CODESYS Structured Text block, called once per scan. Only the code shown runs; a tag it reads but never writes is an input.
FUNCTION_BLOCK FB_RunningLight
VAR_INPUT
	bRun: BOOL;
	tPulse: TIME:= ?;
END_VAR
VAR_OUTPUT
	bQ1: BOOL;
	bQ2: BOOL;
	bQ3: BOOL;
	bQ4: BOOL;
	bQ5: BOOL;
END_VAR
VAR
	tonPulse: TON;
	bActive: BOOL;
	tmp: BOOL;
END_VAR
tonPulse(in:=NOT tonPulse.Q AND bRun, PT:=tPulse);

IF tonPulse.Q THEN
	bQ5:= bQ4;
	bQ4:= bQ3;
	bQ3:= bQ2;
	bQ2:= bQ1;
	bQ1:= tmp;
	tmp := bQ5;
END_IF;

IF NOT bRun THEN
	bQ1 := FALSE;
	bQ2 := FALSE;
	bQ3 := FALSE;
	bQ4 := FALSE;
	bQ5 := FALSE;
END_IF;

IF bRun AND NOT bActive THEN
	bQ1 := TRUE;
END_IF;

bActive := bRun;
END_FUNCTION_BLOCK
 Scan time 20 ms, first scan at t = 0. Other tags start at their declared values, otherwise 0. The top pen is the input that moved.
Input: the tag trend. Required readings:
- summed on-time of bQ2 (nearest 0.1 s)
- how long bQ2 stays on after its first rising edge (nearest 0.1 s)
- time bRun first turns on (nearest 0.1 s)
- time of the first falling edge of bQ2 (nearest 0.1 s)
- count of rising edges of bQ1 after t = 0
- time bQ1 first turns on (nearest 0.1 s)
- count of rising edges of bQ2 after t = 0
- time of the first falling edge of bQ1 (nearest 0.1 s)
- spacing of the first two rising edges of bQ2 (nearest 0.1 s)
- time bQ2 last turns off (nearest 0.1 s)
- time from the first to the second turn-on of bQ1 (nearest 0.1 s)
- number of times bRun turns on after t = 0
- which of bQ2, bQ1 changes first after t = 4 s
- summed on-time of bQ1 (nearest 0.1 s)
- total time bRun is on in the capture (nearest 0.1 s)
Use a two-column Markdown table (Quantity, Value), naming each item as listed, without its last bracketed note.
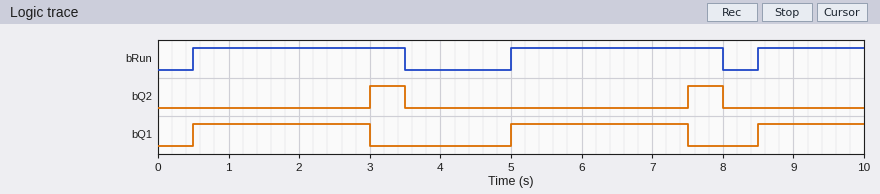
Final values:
| Quantity | Value |
|---|---|
| summed on-time of bQ2 | 1.0 s |
| how long bQ2 stays on after its first rising edge | 0.5 s |
| time bRun first turns on | 0.5 s |
| time of the first falling edge of bQ2 | 3.5 s |
| count of rising edges of bQ1 after t = 0 | 3 |
| time bQ1 first turns on | 0.5 s |
| count of rising edges of bQ2 after t = 0 | 2 |
| time of the first falling edge of bQ1 | 3.0 s |
| spacing of the first two rising edges of bQ2 | 4.5 s |
| time bQ2 last turns off | 8.0 s |
| time from the first to the second turn-on of bQ1 | 4.5 s |
| number of times bRun turns on after t = 0 | 3 |
| which of bQ2, bQ1 changes first after t = 4 s | bQ1 |
| summed on-time of bQ1 | 6.5 s |
| total time bRun is on in the capture | 7.5 s |
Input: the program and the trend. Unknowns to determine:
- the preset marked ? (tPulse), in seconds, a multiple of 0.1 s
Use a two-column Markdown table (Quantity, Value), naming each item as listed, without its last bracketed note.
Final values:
| Quantity | Value |
|---|---|
| the preset marked ? (tPulse), in seconds, a multiple of 0.1 s | 2.5 s |
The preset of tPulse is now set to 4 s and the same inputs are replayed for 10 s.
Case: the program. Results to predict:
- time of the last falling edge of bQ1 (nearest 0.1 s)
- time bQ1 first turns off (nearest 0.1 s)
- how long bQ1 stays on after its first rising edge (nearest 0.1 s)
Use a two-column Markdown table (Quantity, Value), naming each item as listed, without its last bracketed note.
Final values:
| Quantity | Value |
|---|---|
| time of the last falling edge of bQ1 | 8.0 s |
| time bQ1 first turns off | 3.5 s |
| how long bQ1 stays on after its first rising edge | 3.0 s |
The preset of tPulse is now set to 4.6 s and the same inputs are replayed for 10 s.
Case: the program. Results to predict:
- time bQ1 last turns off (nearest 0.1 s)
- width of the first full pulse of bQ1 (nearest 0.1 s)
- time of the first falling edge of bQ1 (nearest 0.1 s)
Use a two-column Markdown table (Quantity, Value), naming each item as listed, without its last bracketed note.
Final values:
| Quantity | Value |
|---|---|
| time bQ1 last turns off | 8.0 s |
| width of the first full pulse of bQ1 | 3.0 s |
| time of the first falling edge of bQ1 | 3.5 s |
